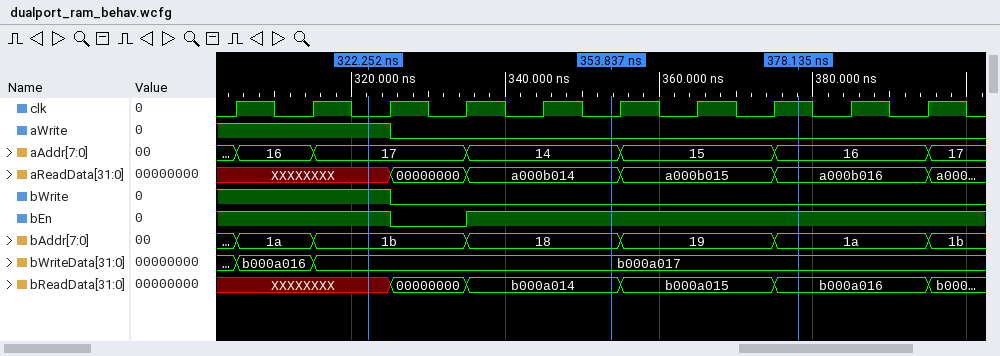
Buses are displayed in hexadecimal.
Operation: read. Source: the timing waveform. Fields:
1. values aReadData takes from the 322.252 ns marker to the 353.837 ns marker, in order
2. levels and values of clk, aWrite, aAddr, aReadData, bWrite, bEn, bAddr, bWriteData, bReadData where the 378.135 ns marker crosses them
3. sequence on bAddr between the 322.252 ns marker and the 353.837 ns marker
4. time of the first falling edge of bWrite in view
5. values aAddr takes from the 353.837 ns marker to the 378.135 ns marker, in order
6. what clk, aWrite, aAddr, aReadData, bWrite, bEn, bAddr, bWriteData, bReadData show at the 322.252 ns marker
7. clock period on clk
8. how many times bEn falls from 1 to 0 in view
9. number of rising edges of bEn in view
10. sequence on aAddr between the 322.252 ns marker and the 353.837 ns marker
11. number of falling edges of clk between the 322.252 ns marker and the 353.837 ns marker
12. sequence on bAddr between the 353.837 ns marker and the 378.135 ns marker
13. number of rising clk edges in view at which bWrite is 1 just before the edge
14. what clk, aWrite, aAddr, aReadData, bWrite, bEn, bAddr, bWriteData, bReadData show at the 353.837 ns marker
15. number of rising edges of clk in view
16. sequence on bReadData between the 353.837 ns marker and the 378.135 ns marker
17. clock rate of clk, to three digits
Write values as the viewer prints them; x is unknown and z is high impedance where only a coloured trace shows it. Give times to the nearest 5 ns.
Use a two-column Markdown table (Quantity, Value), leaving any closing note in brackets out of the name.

| Quantity | Value |
|---|---|
| values aReadData takes from the 322.252 ns marker to the 353.837 ns marker, in order | XXXXXXXX, 00000000, a000b014 |
| levels and values of clk, aWrite, aAddr, aReadData, bWrite, bEn, bAddr, bWriteData, bReadData where the 378.135 ns marker crosses them | clk=1, aWrite=0, aAddr=16, aReadData=a000b016, bWrite=0, bEn=1, bAddr=1a, bWriteData=b000a017, bReadData=b000a016 |
| sequence on bAddr between the 322.252 ns marker and the 353.837 ns marker | 1b, 18 |
| time of the first falling edge of bWrite in view | 325 ns |
| values aAddr takes from the 353.837 ns marker to the 378.135 ns marker, in order | 14, 15, 16 |
| what clk, aWrite, aAddr, aReadData, bWrite, bEn, bAddr, bWriteData, bReadData show at the 322.252 ns marker | clk=0, aWrite=1, aAddr=17, aReadData=XXXXXXXX, bWrite=1, bEn=1, bAddr=1b, bWriteData=b000a017, bReadData=XXXXXXXX |
| clock period on clk | 10 ns |
| how many times bEn falls from 1 to 0 in view | 1 |
| number of rising edges of bEn in view | 1 |
| sequence on aAddr between the 322.252 ns marker and the 353.837 ns marker | 17, 14 |
| number of falling edges of clk between the 322.252 ns marker and the 353.837 ns marker | 3 |
| sequence on bAddr between the 353.837 ns marker and the 378.135 ns marker | 18, 19, 1a |
| number of rising clk edges in view at which bWrite is 1 just before the edge | 3 |
| what clk, aWrite, aAddr, aReadData, bWrite, bEn, bAddr, bWriteData, bReadData show at the 353.837 ns marker | clk=0, aWrite=0, aAddr=14, aReadData=a000b014, bWrite=0, bEn=1, bAddr=18, bWriteData=b000a017, bReadData=b000a014 |
| number of rising edges of clk in view | 10 |
| sequence on bReadData between the 353.837 ns marker and the 378.135 ns marker | b000a014, b000a015, b000a016 |
| clock rate of clk, to three digits | 100 MHz |
